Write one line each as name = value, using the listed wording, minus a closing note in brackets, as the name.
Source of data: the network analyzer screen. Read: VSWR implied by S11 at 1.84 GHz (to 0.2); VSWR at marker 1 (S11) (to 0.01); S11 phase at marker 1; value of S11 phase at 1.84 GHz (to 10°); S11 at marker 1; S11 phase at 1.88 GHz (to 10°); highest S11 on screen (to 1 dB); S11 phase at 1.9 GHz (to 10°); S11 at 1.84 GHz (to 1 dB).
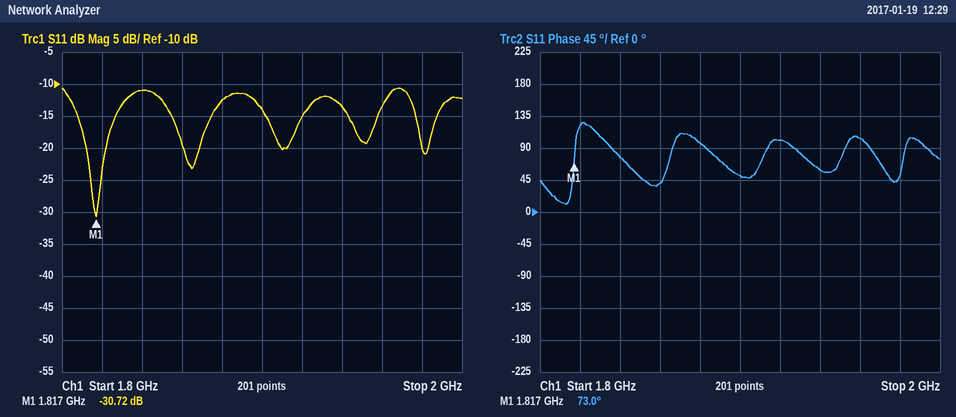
VSWR implied by S11 at 1.84 GHz = 1.8
VSWR at marker 1 (S11) = 1.06
S11 phase at marker 1 = 73.0°
value of S11 phase at 1.84 GHz = 80°
S11 at marker 1 = -30.72 dB
S11 phase at 1.88 GHz = 100°
highest S11 on screen = -11 dB
S11 phase at 1.9 GHz = 50°
S11 at 1.84 GHz = -11 dB
